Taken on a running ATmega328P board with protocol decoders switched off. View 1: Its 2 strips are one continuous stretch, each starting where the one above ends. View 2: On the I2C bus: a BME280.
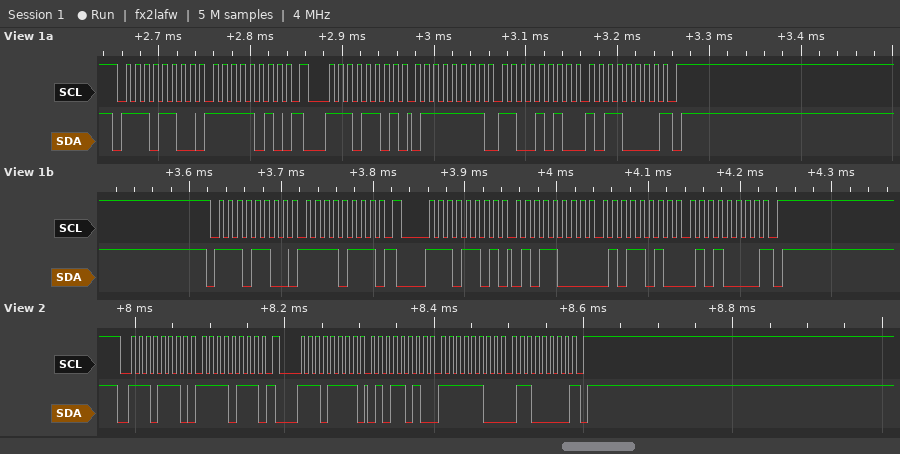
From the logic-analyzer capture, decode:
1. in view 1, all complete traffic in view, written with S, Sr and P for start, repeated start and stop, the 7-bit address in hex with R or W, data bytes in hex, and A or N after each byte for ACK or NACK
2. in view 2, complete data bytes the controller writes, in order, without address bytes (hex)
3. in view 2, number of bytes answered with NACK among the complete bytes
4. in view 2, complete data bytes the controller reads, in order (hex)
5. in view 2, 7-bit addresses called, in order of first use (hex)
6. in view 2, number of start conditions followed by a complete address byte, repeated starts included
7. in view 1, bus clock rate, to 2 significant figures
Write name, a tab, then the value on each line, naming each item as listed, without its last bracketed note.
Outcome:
in view 1, all complete traffic in view, written with S, Sr and P for start, repeated start and stop, the 7-bit address in hex with R or W, data bytes in hex, and A or N after each byte for ACK or NACK	S 76W A FA A Sr 76R A 7F A CA A B0 N P S 76W A F7 A Sr 76R A 58 A 5A A 50 N P
in view 2, complete data bytes the controller writes, in order, without address bytes	F7
in view 2, number of bytes answered with NACK among the complete bytes	1
in view 2, complete data bytes the controller reads, in order	5A FC 60
in view 2, 7-bit addresses called, in order of first use	0x77
in view 2, number of start conditions followed by a complete address byte, repeated starts included	2
in view 1, bus clock rate, to 2 significant figures	100 kHz
